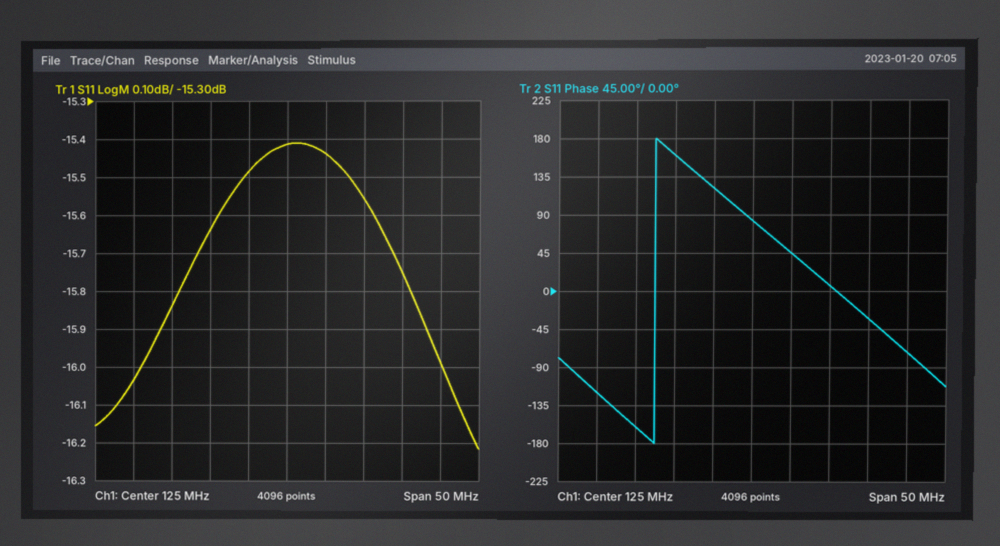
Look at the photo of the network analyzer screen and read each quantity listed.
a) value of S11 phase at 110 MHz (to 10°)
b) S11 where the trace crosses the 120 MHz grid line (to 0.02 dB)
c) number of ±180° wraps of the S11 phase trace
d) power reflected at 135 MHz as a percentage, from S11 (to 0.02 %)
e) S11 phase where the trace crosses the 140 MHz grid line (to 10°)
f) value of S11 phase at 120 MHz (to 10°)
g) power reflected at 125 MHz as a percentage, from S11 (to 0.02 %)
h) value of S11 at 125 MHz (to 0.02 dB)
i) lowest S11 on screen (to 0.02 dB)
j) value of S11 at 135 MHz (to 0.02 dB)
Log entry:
-160°
-15.48 dB
1
2.78 %
-30°
120°
2.88 %
-15.42 dB
-16.22 dB
-15.56 dB
